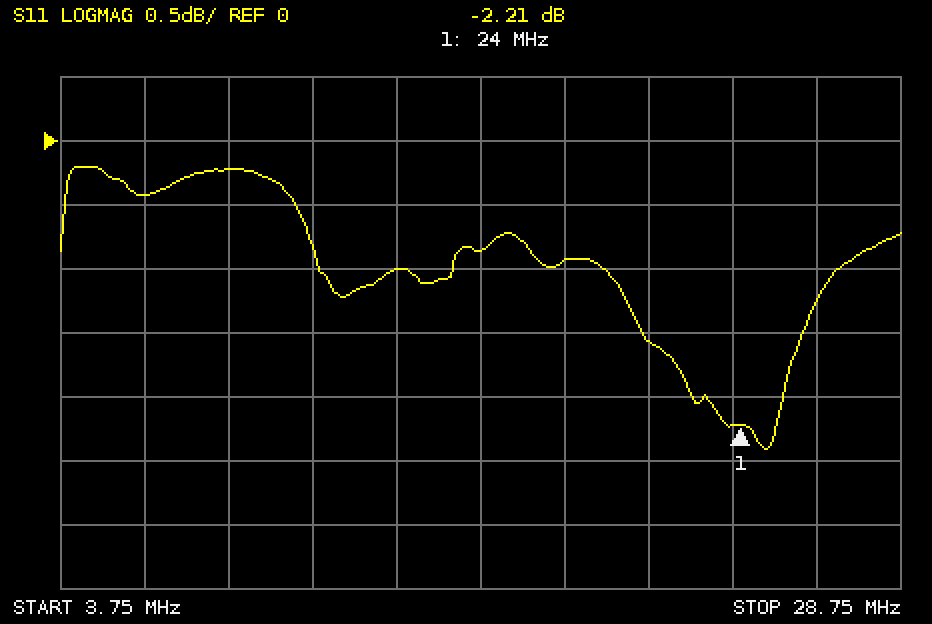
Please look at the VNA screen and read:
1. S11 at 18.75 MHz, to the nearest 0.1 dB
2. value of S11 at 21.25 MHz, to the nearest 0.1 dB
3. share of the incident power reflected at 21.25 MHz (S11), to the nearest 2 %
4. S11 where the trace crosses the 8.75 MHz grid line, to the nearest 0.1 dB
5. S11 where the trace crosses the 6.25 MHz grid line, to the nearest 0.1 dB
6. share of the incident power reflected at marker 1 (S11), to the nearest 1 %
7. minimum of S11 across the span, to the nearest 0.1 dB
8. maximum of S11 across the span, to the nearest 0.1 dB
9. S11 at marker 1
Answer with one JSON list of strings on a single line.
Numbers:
["-0.9 dB", "-1.6 dB", "70 %", "-0.2 dB", "-0.4 dB", "60 %", "-2.4 dB", "-0.2 dB", "-2.21 dB"]
